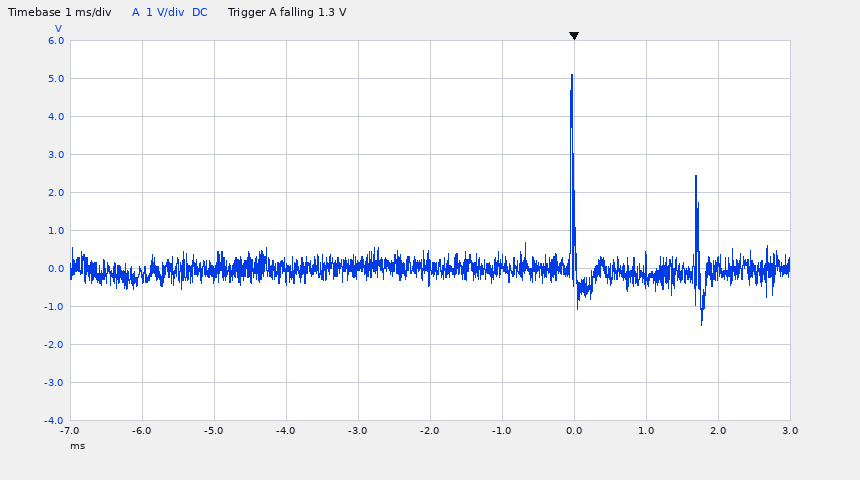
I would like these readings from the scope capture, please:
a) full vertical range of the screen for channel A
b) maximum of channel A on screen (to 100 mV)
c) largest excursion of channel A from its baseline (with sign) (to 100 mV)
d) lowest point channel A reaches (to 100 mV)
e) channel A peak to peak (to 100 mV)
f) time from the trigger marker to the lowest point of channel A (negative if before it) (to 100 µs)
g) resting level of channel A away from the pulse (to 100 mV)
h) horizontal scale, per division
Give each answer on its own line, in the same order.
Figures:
10 V
5.1 V
+5.1 V
-1.5 V
6.6 V
+1.8 ms
0.0 V
1 ms
